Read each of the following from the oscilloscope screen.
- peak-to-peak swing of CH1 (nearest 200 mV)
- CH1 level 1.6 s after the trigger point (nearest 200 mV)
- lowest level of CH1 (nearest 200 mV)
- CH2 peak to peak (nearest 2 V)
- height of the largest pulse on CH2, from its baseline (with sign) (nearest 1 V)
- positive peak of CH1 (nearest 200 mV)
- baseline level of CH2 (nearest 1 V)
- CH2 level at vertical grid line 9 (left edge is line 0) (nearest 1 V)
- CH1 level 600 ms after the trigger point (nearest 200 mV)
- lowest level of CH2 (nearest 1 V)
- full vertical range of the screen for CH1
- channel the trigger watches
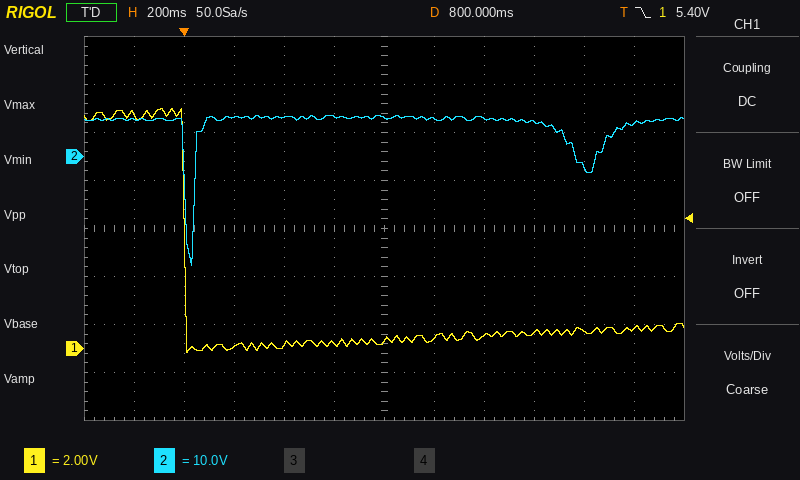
10.2 V
800 mV
-200 mV
32 V
-31 V
10.0 V
8 V
7 V
200 mV
-23 V
16 V
CH1
